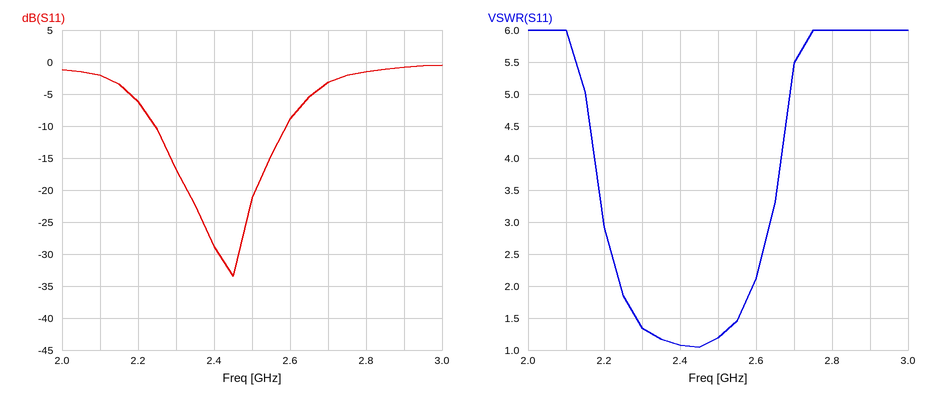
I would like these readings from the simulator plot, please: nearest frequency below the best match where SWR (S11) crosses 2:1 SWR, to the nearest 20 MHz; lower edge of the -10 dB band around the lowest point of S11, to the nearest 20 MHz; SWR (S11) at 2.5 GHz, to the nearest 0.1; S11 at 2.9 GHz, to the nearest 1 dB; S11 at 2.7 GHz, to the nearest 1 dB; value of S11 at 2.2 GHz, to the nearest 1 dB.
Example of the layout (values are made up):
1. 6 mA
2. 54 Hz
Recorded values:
1. 2.24 GHz
2. 2.24 GHz
3. 1.2
4. -1 dB
5. -3 dB
6. -6 dB
